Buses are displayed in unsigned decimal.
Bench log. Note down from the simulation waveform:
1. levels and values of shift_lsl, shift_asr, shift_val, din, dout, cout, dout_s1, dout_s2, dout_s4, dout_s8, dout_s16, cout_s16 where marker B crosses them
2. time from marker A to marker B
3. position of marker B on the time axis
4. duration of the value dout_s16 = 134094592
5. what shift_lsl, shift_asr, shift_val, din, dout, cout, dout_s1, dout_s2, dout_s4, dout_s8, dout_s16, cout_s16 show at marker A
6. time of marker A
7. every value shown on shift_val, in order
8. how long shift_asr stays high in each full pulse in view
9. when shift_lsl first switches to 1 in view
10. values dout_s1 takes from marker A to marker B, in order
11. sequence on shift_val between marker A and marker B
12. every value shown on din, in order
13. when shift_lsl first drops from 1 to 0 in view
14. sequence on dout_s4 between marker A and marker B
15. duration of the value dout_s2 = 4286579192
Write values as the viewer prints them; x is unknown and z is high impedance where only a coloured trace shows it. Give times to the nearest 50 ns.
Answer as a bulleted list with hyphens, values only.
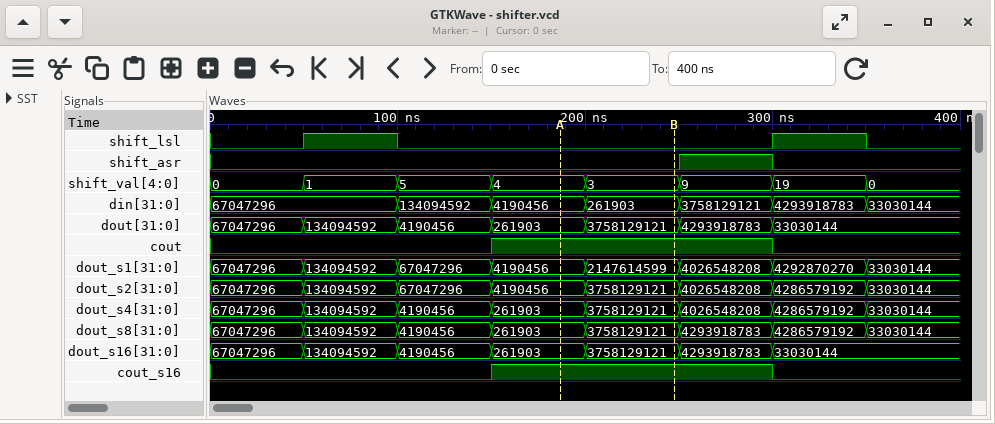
- shift_lsl=0, shift_asr=0, shift_val=3, din=261903, dout=3758129121, cout=1, dout_s1=2147614599, dout_s2=3758129121, dout_s4=3758129121, dout_s8=3758129121, dout_s16=3758129121, cout_s16=1
- 50 ns
- 250 ns
- 50 ns
- shift_lsl=0, shift_asr=0, shift_val=4, din=4190456, dout=261903, cout=1, dout_s1=4190456, dout_s2=4190456, dout_s4=261903, dout_s8=261903, dout_s16=261903, cout_s16=1
- 200 ns
- 0, 1, 5, 4, 3, 9, 19, 0
- 50 ns
- 50 ns
- 4190456, 2147614599
- 4, 3
- 67047296, 134094592, 4190456, 261903, 3758129121, 4293918783, 33030144
- 100 ns
- 261903, 3758129121
- 50 ns
